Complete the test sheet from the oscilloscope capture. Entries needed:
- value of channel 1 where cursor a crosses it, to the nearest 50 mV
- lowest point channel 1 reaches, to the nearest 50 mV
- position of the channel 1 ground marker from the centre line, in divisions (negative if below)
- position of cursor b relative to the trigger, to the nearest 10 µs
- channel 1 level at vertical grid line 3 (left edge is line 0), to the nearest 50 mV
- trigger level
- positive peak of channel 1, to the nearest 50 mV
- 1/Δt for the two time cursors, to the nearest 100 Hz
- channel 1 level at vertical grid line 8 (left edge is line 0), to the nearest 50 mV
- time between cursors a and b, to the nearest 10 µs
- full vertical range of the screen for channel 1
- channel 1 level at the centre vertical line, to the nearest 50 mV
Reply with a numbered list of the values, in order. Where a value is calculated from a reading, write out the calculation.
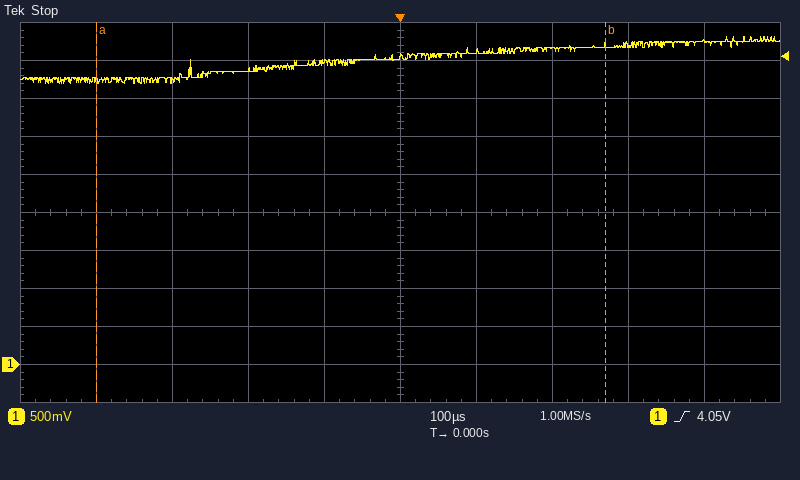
1. 3.75 V
2. 3.70 V
3. -4.0 div
4. +270 µs
5. 3.90 V
6. 4.05 V
7. 4.30 V
8. 1 / 670 µs ≈ 1.5 kHz
9. 4.20 V
10. 670 µs
11. 5 V
12. 4.05 V
